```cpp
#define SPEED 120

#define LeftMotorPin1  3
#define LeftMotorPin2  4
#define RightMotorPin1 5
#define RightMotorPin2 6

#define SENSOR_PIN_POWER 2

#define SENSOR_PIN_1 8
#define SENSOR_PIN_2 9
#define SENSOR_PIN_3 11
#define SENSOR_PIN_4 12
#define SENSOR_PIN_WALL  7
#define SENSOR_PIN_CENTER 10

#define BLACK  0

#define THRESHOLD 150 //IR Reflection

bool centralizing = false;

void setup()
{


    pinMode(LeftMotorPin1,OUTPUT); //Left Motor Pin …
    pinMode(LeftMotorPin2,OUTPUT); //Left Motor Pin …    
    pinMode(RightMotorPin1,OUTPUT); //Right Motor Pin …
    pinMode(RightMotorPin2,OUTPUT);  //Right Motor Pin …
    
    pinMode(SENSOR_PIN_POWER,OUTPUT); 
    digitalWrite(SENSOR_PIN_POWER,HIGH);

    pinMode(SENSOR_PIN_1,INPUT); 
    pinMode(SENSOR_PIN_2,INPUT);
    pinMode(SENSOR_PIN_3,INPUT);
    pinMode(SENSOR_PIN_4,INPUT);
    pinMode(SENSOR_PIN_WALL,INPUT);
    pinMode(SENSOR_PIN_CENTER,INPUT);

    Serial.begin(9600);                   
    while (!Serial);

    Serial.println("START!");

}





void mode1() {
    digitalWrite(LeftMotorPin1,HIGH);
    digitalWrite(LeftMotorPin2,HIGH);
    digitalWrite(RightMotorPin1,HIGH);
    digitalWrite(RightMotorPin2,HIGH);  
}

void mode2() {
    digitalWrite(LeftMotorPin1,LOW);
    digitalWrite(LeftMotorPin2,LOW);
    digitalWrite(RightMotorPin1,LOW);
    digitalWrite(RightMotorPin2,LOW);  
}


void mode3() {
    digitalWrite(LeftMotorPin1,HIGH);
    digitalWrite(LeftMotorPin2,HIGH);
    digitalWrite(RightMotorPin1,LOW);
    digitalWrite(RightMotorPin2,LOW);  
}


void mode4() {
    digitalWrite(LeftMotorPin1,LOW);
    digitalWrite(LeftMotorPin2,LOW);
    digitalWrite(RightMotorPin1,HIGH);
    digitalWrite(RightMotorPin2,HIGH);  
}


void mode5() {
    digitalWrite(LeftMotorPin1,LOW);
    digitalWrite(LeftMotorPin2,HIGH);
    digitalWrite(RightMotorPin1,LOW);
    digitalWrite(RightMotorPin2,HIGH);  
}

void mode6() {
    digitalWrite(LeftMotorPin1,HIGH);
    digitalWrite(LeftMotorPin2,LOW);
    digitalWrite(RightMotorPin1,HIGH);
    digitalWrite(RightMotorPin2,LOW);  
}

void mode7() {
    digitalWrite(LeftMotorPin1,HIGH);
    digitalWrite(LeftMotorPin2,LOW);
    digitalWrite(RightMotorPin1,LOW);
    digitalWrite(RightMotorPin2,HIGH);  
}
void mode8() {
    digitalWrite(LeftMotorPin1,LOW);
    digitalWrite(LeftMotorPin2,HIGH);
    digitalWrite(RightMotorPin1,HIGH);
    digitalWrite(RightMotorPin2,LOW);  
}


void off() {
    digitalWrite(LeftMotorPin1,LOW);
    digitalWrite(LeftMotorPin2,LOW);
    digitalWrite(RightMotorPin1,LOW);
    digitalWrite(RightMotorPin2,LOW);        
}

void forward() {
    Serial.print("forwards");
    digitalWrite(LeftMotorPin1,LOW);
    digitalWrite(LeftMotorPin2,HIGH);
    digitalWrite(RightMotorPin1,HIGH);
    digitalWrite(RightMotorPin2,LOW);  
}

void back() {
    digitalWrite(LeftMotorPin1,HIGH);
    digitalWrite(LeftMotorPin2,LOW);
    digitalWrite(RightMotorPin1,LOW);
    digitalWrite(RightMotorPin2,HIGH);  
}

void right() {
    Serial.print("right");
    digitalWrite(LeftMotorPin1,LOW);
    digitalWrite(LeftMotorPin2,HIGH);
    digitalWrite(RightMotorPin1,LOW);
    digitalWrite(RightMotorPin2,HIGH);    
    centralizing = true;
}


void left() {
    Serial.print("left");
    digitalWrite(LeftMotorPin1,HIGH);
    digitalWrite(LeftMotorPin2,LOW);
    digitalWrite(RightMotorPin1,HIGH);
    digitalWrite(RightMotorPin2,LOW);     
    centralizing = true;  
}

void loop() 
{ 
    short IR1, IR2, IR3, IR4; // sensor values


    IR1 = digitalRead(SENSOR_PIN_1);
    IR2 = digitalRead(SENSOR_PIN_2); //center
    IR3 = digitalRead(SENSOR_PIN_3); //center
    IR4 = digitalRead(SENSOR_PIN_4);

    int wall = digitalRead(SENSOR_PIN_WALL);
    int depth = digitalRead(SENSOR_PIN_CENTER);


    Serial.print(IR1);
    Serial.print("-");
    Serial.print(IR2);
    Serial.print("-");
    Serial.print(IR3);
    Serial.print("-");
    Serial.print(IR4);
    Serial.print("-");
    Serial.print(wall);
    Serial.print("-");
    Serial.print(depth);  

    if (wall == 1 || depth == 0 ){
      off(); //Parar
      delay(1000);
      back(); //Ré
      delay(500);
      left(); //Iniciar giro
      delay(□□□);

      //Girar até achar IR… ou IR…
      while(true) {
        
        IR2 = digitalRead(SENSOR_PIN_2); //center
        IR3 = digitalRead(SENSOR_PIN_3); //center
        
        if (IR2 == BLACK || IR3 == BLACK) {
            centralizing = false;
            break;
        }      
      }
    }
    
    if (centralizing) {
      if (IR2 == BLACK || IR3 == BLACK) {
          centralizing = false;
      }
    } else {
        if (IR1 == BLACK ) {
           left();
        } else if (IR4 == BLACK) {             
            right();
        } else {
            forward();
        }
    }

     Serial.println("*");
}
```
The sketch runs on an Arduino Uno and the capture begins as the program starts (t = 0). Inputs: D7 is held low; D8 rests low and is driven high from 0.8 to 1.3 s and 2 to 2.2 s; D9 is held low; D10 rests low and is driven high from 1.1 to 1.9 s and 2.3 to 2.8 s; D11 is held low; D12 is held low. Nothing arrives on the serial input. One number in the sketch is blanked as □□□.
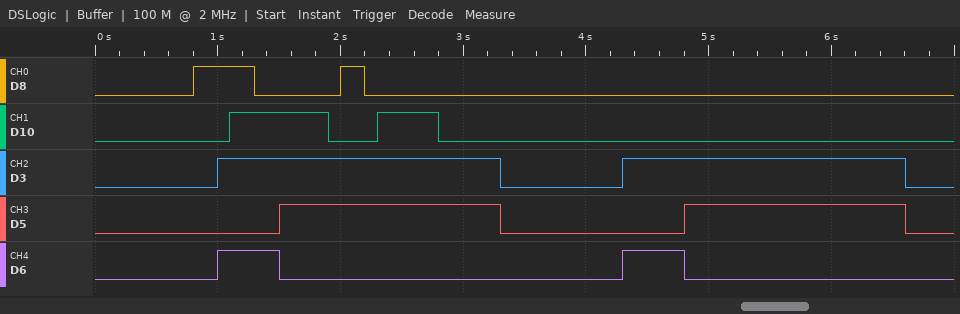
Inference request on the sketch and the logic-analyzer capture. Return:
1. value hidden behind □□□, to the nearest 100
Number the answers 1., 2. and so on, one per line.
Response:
1. 1800
